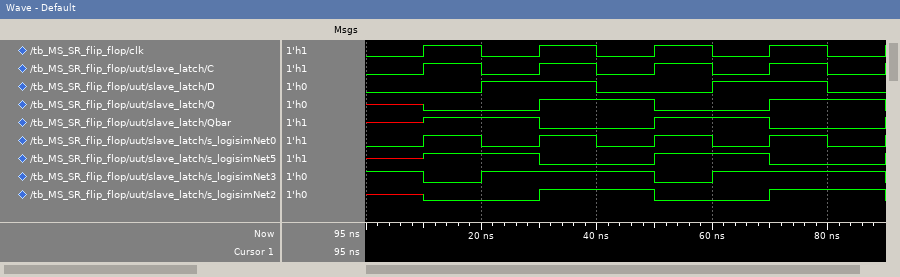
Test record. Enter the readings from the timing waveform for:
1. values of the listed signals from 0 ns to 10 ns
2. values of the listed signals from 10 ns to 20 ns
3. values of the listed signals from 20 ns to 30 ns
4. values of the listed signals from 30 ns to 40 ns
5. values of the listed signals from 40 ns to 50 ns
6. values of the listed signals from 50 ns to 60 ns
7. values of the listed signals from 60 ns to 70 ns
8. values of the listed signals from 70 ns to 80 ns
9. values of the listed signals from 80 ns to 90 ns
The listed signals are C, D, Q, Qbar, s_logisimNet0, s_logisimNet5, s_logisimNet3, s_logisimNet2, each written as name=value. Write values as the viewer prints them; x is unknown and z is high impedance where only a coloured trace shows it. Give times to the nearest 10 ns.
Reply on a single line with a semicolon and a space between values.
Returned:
C=0, D=0, Q=x, Qbar=x, s_logisimNet0=0, s_logisimNet5=x, s_logisimNet3=1, s_logisimNet2=x; C=1, D=0, Q=0, Qbar=1, s_logisimNet0=1, s_logisimNet5=1, s_logisimNet3=0, s_logisimNet2=0; C=0, D=1, Q=0, Qbar=1, s_logisimNet0=0, s_logisimNet5=1, s_logisimNet3=1, s_logisimNet2=0; C=1, D=1, Q=1, Qbar=0, s_logisimNet0=1, s_logisimNet5=0, s_logisimNet3=1, s_logisimNet2=1; C=0, D=0, Q=1, Qbar=0, s_logisimNet0=0, s_logisimNet5=0, s_logisimNet3=1, s_logisimNet2=1; C=1, D=0, Q=0, Qbar=1, s_logisimNet0=1, s_logisimNet5=1, s_logisimNet3=0, s_logisimNet2=0; C=0, D=1, Q=0, Qbar=1, s_logisimNet0=0, s_logisimNet5=1, s_logisimNet3=1, s_logisimNet2=0; C=1, D=1, Q=1, Qbar=0, s_logisimNet0=1, s_logisimNet5=0, s_logisimNet3=1, s_logisimNet2=1; C=0, D=0, Q=1, Qbar=0, s_logisimNet0=0, s_logisimNet5=0, s_logisimNet3=1, s_logisimNet2=1
